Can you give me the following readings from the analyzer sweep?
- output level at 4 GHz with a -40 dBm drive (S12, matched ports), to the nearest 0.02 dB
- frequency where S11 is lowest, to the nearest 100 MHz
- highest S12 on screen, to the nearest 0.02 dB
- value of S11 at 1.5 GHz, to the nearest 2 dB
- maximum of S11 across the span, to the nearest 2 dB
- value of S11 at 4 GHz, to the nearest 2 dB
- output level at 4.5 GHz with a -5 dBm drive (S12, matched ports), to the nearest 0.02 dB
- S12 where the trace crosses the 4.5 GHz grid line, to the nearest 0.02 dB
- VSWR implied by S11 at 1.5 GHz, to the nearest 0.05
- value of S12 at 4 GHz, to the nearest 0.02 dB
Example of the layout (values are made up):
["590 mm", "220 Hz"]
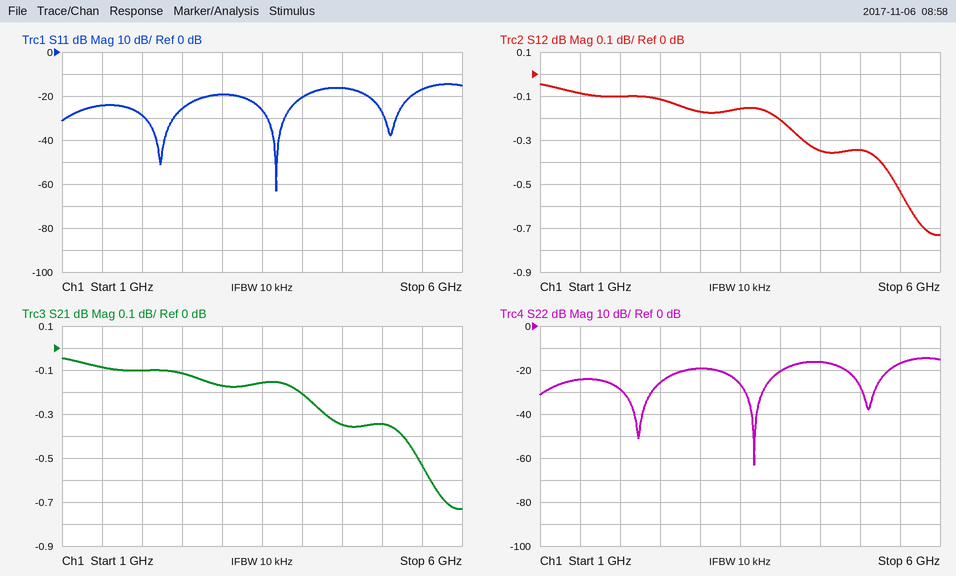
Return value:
["-40.20 dBm", "3.7 GHz", "-0.04 dB", "-24 dB", "-14 dB", "-20 dB", "-5.34 dBm", "-0.34 dB", "1.15", "-0.20 dB"]
